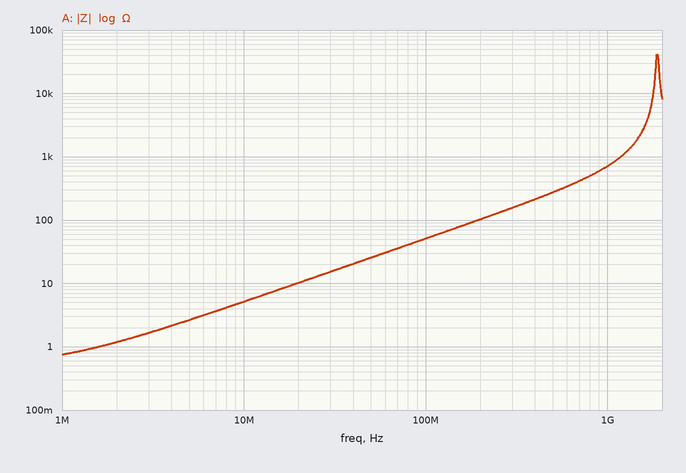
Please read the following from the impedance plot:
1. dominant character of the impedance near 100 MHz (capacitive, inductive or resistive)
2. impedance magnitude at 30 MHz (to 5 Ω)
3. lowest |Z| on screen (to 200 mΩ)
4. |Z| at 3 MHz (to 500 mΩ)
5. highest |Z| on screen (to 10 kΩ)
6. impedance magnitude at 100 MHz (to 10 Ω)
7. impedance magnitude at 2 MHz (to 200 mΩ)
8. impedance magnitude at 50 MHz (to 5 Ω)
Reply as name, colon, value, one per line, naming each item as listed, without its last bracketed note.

dominant character of the impedance near 100 MHz: inductive
impedance magnitude at 30 MHz: 15 Ω
lowest |Z| on screen: 800 mΩ
|Z| at 3 MHz: 1.5 Ω
highest |Z| on screen: 40 kΩ
impedance magnitude at 100 MHz: 50 Ω
impedance magnitude at 2 MHz: 1.2 Ω
impedance magnitude at 50 MHz: 25 Ω
